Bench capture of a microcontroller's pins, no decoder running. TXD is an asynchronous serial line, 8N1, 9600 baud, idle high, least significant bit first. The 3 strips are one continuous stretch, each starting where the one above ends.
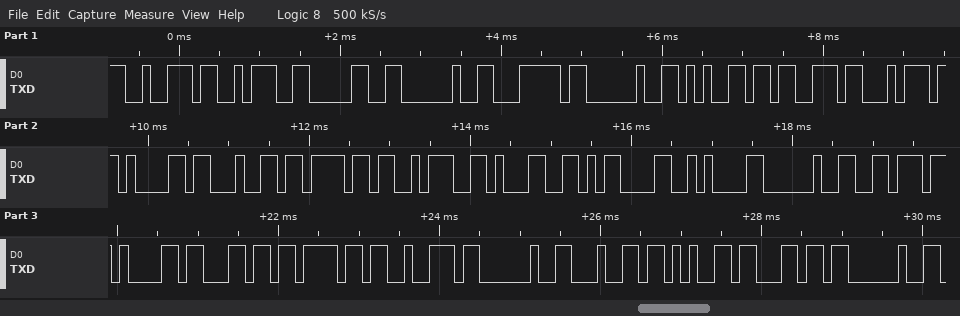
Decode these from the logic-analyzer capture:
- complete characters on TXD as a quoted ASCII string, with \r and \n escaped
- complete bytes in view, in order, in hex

"r:0 | estado:1\r\n valor del "
72 3A 30 20 7C 20 65 73 74 61 64 6F 3A 31 0D 0A 20 76 61 6C 6F 72 20 64 65 6C 20
